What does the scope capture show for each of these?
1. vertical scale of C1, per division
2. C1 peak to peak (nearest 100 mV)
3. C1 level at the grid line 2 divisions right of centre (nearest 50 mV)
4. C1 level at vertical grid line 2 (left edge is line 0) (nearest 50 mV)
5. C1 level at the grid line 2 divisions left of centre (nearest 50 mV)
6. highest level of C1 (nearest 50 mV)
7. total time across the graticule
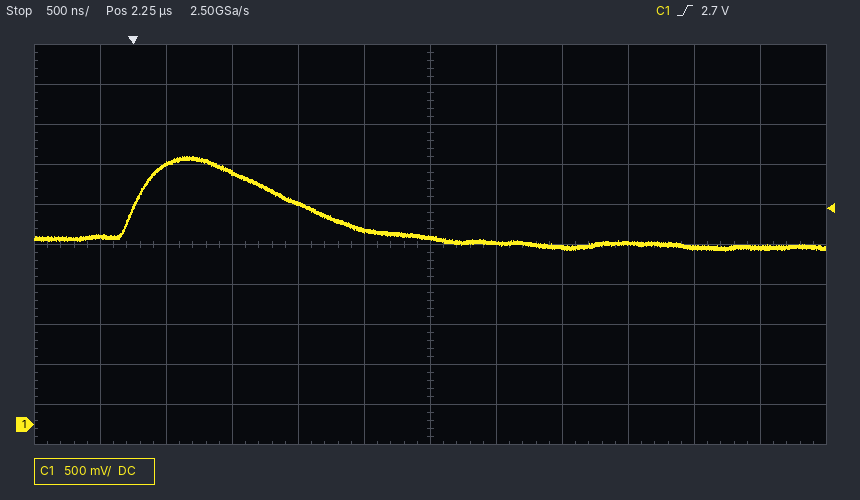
500 mV
1.20 V
2.20 V
3.25 V
2.75 V
3.35 V
6 µs
